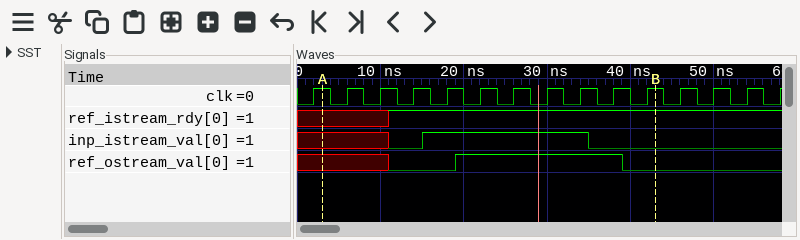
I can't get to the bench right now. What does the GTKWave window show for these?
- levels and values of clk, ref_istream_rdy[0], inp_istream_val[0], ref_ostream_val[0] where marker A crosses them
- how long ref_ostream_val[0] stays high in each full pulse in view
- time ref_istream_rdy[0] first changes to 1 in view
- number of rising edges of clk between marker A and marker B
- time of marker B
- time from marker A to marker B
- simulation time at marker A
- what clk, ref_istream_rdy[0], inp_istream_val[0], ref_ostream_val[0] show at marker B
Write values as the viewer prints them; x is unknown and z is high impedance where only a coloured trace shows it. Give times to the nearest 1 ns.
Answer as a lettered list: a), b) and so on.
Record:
a) clk=1, ref_istream_rdy[0]=x, inp_istream_val[0]=x, ref_ostream_val[0]=x
b) 20 ns
c) 11 ns
d) 10
e) 43 ns
f) 40 ns
g) 3 ns
h) clk=1, ref_istream_rdy[0]=1, inp_istream_val[0]=0, ref_ostream_val[0]=0
